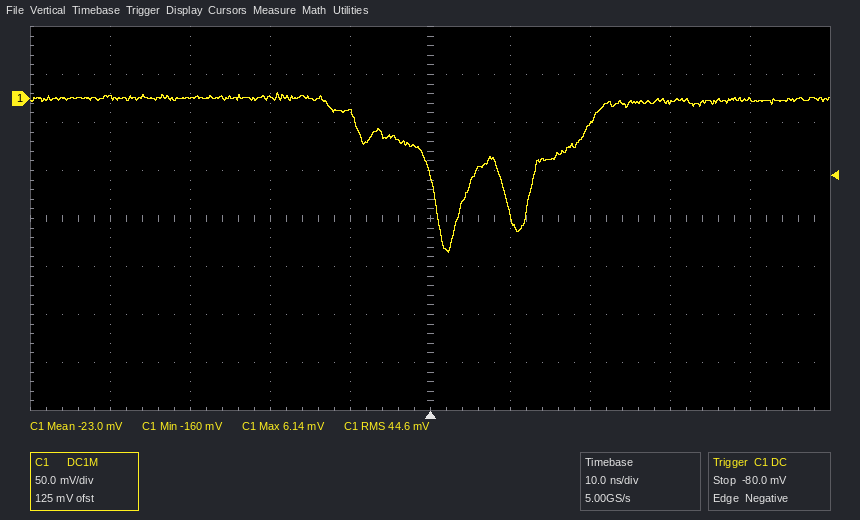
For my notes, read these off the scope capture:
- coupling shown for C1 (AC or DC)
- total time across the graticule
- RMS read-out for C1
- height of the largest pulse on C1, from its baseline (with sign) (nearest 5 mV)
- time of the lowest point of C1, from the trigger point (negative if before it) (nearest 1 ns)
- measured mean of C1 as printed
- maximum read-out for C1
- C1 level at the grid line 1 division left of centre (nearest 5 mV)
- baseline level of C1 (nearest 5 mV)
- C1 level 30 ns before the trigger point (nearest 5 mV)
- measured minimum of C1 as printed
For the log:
DC
100 ns
44.6 mV
-160 mV
+2 ns
-23.0 mV
6.14 mV
-15 mV
0 mV
0 mV
-160 mV
